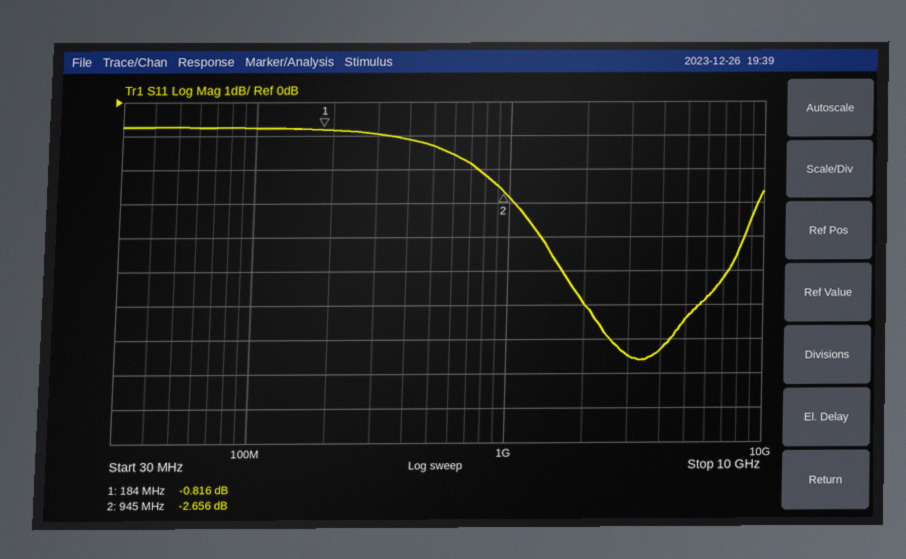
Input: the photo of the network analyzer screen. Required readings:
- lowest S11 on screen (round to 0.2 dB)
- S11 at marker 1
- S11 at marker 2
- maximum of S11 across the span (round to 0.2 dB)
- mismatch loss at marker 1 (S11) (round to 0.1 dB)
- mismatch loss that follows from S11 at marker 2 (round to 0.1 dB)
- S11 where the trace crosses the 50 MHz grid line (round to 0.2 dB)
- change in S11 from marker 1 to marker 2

-7.6 dB
-0.816 dB
-2.656 dB
-0.8 dB
7.7 dB
3.4 dB
-0.8 dB
-1.840 dB
